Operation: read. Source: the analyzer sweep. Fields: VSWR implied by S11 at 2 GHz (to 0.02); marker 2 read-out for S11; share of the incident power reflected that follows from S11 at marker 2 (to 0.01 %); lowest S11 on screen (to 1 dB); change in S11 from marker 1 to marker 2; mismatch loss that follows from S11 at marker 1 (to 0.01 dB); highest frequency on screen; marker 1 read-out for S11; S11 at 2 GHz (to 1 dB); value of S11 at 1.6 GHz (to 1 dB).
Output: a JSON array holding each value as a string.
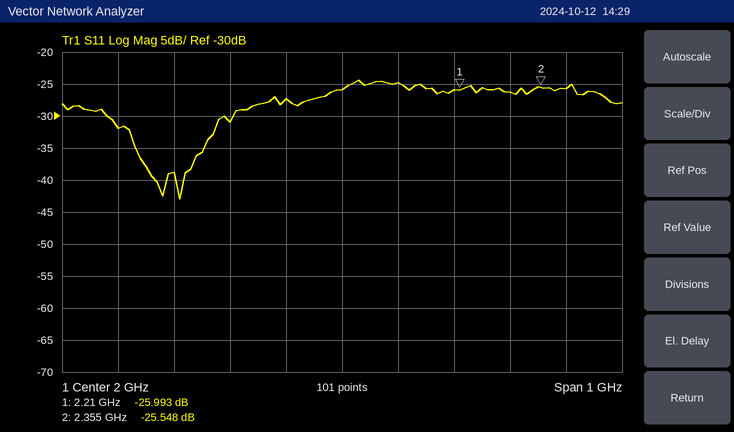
["1.10", "-25.548 dB", "0.28 %", "-43 dB", "0.445 dB", "0.01 dB", "2.5 GHz", "-25.993 dB", "-26 dB", "-32 dB"]
